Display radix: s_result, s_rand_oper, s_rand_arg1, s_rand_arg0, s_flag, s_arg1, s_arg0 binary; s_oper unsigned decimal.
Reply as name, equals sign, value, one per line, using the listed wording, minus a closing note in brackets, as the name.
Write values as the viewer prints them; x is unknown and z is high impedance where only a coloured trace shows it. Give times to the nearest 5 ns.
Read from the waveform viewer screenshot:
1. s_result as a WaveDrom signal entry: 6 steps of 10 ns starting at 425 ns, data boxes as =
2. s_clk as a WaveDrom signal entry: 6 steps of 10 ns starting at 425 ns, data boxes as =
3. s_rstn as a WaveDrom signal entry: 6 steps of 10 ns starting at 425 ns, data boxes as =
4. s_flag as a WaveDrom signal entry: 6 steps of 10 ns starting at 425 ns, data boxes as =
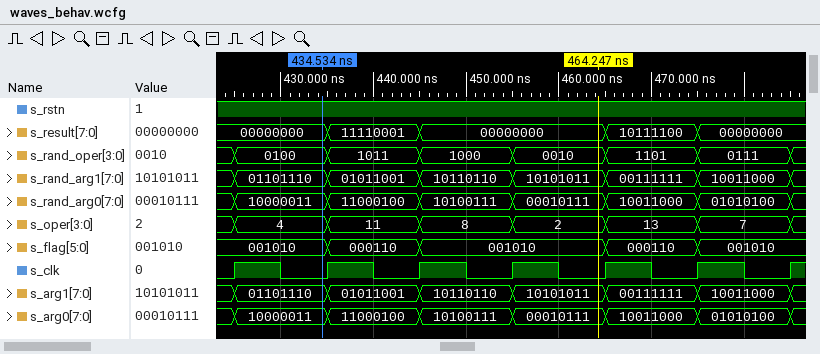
s_result as a WaveDrom signal entry: 6 steps of 10 ns starting at 425 ns, data boxes as = = {name: 's_result', wave: '===.==', data: '00000000 11110001 00000000 10111100 00000000'}
s_clk as a WaveDrom signal entry: 6 steps of 10 ns starting at 425 ns, data boxes as = = {name: 's_clk', wave: 'p.....'}
s_rstn as a WaveDrom signal entry: 6 steps of 10 ns starting at 425 ns, data boxes as = = {name: 's_rstn', wave: '1.....'}
s_flag as a WaveDrom signal entry: 6 steps of 10 ns starting at 425 ns, data boxes as = = {name: 's_flag', wave: '===.==', data: '001010 000110 001010 000110 001010'}
